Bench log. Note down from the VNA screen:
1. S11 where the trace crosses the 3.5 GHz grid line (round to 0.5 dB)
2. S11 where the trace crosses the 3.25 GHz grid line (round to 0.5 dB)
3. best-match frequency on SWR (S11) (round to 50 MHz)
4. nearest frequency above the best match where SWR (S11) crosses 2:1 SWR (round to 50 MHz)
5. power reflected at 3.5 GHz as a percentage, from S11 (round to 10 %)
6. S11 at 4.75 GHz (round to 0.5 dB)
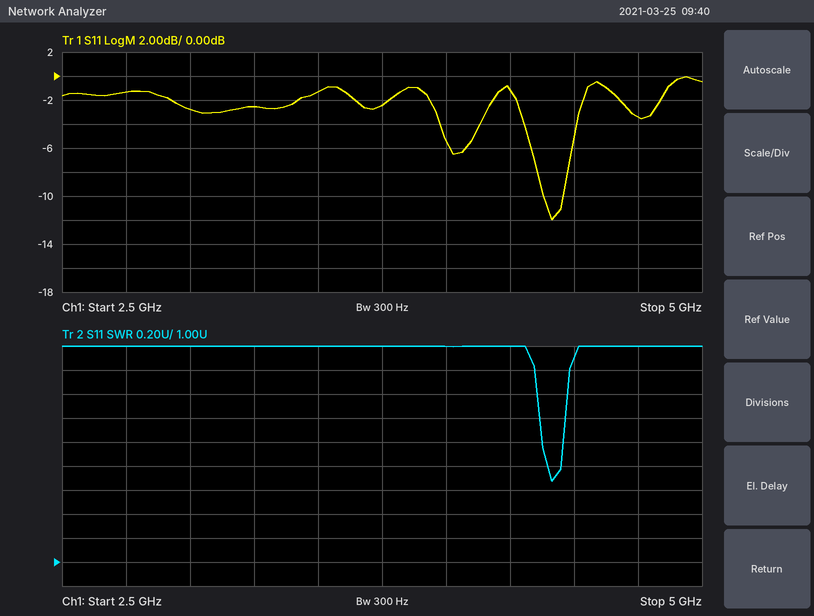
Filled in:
-1.5 dB
-2.5 dB
4.40 GHz
4.45 GHz
70 %
-3.5 dB
